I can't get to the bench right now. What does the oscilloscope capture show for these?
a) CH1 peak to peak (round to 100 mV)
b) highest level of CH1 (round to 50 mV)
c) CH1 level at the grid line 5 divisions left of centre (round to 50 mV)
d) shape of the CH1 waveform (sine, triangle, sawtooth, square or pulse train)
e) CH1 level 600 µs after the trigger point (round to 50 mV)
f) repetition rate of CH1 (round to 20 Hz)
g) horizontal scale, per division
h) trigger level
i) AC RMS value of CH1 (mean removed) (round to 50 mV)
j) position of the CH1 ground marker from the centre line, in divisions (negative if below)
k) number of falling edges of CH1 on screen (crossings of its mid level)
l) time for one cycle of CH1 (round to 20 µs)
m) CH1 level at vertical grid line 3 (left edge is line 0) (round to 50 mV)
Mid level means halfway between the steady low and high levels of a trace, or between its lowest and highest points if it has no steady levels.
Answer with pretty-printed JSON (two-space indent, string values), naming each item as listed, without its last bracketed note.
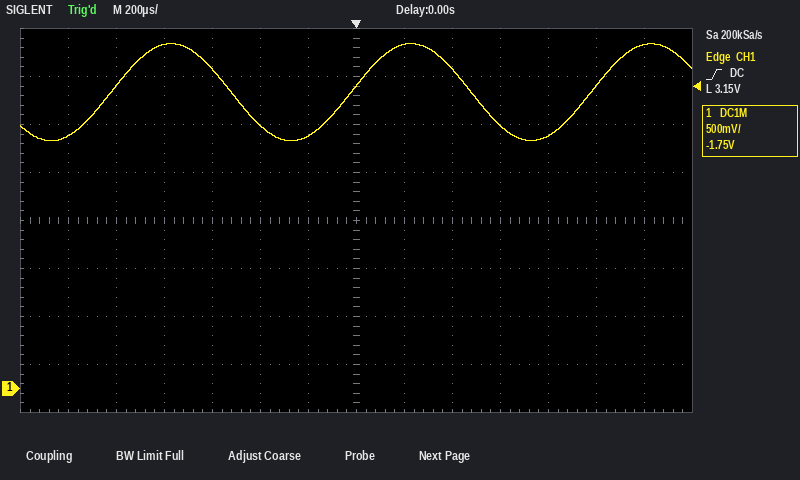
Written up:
{
  "CH1 peak to peak": "1.00 V",
  "highest level of CH1": "3.60 V",
  "CH1 level at the grid line 5 divisions left of centre": "3.15 V",
  "shape of the CH1 waveform": "sine",
  "CH1 level 600 µs after the trigger point": "2.75 V",
  "repetition rate of CH1": "1.00 kHz",
  "horizontal scale, per division": "200 µs",
  "trigger level": "3.15 V",
  "AC RMS value of CH1 (mean removed)": "350 mV",
  "position of the CH1 ground marker from the centre line, in divisions": "-3.5 div",
  "number of falling edges of CH1 on screen": "2",
  "time for one cycle of CH1": "1.00 ms",
  "CH1 level at vertical grid line 3 (left edge is line 0)": "3.60 V"
}
